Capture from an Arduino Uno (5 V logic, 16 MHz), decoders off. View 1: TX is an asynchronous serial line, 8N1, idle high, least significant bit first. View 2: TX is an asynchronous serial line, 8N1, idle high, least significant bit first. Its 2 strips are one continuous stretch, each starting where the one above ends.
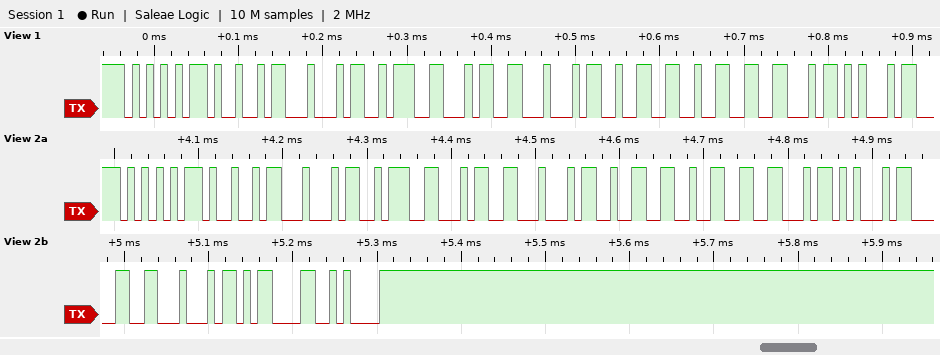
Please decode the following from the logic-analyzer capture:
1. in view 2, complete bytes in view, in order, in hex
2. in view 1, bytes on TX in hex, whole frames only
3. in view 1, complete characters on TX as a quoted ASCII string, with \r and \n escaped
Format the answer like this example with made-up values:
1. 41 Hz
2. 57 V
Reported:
1. 55 49 44 3A 34 44 32 32 46 45 30 44 0D 0A
2. 0x55 0x49 0x44 0x3A 0x34 0x44 0x32 0x32 0x46 0x45
3. "UID:4D22FE"
